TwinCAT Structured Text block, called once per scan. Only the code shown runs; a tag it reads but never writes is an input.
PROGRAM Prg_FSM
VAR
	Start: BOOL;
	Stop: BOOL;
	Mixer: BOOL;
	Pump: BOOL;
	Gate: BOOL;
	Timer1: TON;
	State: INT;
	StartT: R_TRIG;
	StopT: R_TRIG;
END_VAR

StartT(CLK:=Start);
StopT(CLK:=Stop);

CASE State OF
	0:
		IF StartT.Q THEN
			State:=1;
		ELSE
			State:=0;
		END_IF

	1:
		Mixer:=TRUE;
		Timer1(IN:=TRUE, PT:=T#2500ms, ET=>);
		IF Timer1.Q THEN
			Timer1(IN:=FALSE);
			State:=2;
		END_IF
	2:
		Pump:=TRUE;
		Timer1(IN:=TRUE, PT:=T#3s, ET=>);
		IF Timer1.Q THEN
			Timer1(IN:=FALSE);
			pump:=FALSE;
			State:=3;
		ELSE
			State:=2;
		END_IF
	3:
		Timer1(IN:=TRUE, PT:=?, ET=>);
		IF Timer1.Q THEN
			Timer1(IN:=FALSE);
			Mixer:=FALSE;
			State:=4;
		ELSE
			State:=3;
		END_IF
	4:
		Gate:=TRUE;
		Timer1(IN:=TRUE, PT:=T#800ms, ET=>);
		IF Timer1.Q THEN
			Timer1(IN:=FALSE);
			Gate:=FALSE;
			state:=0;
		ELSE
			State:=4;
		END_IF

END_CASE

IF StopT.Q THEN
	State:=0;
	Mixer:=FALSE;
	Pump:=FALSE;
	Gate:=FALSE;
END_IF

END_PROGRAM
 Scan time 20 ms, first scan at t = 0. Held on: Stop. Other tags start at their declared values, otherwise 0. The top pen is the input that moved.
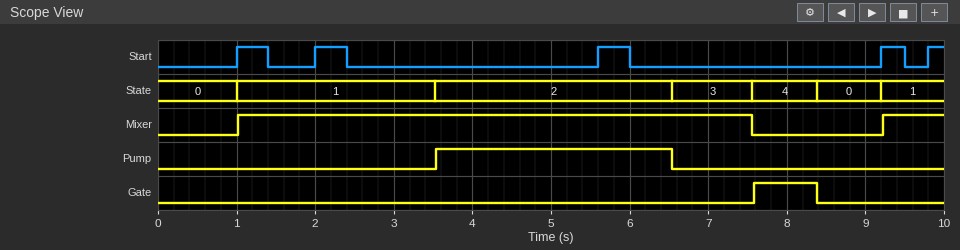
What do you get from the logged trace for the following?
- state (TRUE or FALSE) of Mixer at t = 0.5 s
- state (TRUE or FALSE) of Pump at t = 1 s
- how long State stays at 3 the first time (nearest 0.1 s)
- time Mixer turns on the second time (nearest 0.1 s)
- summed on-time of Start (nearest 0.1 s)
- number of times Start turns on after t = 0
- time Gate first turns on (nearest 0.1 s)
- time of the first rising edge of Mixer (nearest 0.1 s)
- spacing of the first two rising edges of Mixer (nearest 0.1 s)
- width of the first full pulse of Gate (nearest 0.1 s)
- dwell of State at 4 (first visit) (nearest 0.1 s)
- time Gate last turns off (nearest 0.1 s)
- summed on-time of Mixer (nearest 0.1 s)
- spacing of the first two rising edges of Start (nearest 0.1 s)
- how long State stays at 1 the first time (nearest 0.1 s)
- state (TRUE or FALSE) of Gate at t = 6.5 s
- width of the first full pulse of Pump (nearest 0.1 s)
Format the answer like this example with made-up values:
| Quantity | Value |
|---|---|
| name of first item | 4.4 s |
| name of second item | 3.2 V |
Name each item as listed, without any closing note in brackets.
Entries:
| Quantity | Value |
|---|---|
| state (TRUE or FALSE) of Mixer at t = 0.5 s | FALSE |
| state (TRUE or FALSE) of Pump at t = 1 s | FALSE |
| how long State stays at 3 the first time | 1.0 s |
| time Mixer turns on the second time | 9.2 s |
| summed on-time of Start | 1.7 s |
| number of times Start turns on after t = 0 | 5 |
| time Gate first turns on | 7.6 s |
| time of the first rising edge of Mixer | 1.0 s |
| spacing of the first two rising edges of Mixer | 8.2 s |
| width of the first full pulse of Gate | 0.8 s |
| dwell of State at 4 (first visit) | 0.8 s |
| time Gate last turns off | 8.4 s |
| summed on-time of Mixer | 7.3 s |
| spacing of the first two rising edges of Start | 1.0 s |
| how long State stays at 1 the first time | 2.5 s |
| state (TRUE or FALSE) of Gate at t = 6.5 s | FALSE |
| width of the first full pulse of Pump | 3.0 s |
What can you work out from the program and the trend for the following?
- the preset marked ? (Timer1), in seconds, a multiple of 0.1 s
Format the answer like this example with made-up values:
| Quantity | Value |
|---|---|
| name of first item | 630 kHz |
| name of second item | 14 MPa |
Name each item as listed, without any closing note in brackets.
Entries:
| Quantity | Value |
|---|---|
| the preset marked ? (Timer1), in seconds, a multiple of 0.1 s | 1.0 s |
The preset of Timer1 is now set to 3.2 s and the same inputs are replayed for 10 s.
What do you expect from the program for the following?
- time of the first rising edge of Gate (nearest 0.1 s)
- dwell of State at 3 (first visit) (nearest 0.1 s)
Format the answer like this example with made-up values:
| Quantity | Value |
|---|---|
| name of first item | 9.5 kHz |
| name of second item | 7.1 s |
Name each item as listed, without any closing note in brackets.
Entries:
| Quantity | Value |
|---|---|
| time of the first rising edge of Gate | 9.8 s |
| dwell of State at 3 (first visit) | 3.2 s |
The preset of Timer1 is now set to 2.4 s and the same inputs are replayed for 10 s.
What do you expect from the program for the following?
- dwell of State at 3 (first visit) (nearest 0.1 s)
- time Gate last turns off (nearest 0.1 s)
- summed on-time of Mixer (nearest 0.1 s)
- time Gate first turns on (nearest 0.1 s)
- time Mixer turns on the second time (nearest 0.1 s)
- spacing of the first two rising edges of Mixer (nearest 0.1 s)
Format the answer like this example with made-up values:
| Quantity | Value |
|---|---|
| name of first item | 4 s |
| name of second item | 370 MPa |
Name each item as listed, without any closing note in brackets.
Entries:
| Quantity | Value |
|---|---|
| dwell of State at 3 (first visit) | 2.4 s |
| time Gate last turns off | 9.8 s |
| summed on-time of Mixer | 8.1 s |
| time Gate first turns on | 9.0 s |
| time Mixer turns on the second time | 9.8 s |
| spacing of the first two rising edges of Mixer | 8.8 s |
